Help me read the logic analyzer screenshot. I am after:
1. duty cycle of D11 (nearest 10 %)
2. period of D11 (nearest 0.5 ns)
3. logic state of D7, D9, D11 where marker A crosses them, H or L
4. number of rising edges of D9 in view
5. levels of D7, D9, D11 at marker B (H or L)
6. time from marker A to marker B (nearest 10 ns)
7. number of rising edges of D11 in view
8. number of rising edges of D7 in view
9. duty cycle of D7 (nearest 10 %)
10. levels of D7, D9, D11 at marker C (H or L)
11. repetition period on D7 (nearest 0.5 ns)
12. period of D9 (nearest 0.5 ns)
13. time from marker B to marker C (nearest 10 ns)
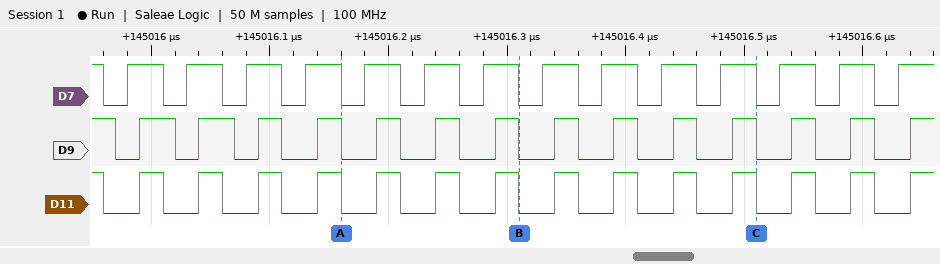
40 %
50 ns
D7=L, D9=L, D11=L
14
D7=L, D9=L, D11=L
150 ns
14
14
60 %
D7=L, D9=L, D11=L
50 ns
50 ns
200 ns
